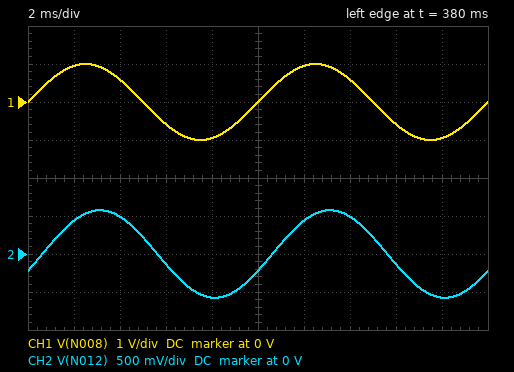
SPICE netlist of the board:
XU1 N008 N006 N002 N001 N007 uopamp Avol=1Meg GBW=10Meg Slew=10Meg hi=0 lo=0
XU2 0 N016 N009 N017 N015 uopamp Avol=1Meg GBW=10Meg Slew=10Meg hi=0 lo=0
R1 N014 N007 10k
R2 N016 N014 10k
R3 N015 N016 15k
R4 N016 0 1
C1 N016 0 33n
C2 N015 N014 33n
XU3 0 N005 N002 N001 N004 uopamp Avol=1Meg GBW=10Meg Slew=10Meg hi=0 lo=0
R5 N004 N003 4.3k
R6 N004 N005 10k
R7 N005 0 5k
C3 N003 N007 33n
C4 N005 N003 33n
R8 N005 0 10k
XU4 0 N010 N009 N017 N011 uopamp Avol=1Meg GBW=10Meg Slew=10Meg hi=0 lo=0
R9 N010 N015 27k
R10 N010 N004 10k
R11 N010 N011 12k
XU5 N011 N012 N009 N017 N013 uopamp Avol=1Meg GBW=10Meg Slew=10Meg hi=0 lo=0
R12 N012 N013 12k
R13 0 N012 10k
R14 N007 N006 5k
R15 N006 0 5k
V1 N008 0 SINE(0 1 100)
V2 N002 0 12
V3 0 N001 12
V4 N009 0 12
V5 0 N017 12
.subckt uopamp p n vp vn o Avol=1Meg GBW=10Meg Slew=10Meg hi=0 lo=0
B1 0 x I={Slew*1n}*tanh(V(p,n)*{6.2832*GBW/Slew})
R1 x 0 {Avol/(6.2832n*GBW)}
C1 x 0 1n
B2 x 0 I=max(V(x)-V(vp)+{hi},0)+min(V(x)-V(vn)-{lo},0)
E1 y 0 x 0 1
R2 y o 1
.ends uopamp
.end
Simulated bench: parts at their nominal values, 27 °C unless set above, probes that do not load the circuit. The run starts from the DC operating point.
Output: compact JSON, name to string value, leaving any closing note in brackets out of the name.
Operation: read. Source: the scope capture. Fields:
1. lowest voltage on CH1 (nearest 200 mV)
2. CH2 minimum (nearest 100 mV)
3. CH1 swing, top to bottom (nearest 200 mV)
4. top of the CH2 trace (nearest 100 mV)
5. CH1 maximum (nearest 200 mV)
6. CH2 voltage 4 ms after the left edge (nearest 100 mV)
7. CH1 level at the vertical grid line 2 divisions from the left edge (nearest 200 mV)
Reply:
{"lowest voltage on CH1": "-1.0 V", "CH2 minimum": "-600 mV", "CH1 swing, top to bottom": "2.0 V", "top of the CH2 trace": "600 mV", "CH1 maximum": "1.0 V", "CH2 voltage 4 ms after the left edge": "500 mV", "CH1 level at the vertical grid line 2 divisions from the left edge": "600 mV"}
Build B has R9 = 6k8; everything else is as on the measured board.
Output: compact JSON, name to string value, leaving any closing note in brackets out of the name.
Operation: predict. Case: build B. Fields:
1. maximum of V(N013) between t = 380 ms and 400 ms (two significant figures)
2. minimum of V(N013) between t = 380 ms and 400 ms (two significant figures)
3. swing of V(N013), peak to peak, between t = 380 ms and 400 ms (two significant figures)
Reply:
{"maximum of V(N013) between t = 380 ms and 400 ms": "5.3 V", "minimum of V(N013) between t = 380 ms and 400 ms": "-5.3 V", "swing of V(N013), peak to peak, between t = 380 ms and 400 ms": "11 V"}
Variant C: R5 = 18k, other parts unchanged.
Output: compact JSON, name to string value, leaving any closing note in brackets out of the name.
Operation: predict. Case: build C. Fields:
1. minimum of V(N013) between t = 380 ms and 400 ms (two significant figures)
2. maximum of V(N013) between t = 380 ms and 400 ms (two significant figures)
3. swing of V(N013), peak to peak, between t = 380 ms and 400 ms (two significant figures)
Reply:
{"minimum of V(N013) between t = 380 ms and 400 ms": "-1.1 V", "maximum of V(N013) between t = 380 ms and 400 ms": "1.1 V", "swing of V(N013), peak to peak, between t = 380 ms and 400 ms": "2.2 V"}
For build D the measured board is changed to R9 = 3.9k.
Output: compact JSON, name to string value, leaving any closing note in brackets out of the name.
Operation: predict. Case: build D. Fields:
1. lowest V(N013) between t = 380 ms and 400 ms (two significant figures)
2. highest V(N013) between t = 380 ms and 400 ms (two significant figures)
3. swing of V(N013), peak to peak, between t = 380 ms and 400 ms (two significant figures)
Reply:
{"lowest V(N013) between t = 380 ms and 400 ms": "-9.3 V", "highest V(N013) between t = 380 ms and 400 ms": "9.3 V", "swing of V(N013), peak to peak, between t = 380 ms and 400 ms": "19 V"}
